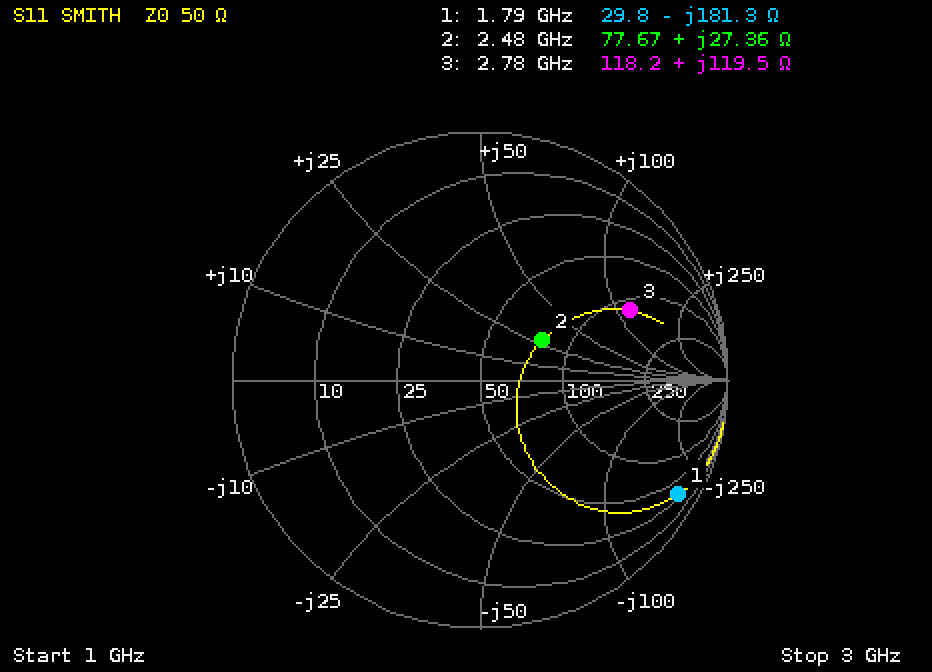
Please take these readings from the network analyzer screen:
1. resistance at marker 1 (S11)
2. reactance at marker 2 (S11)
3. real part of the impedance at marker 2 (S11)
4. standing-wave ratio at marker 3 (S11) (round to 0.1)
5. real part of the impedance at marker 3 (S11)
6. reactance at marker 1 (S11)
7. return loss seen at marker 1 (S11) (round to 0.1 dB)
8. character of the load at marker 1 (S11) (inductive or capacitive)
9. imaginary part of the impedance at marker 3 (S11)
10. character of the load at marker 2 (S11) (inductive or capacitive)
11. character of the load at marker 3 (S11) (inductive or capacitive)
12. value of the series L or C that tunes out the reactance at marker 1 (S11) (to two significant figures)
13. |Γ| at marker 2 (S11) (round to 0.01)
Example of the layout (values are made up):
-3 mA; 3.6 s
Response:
29.8 Ω; +27.36 Ω; 77.67 Ω; 5.0; 118.2 Ω; -181.3 Ω; 0.7 dB; capacitive; +119.5 Ω; inductive; inductive; 16 nH; 0.30
